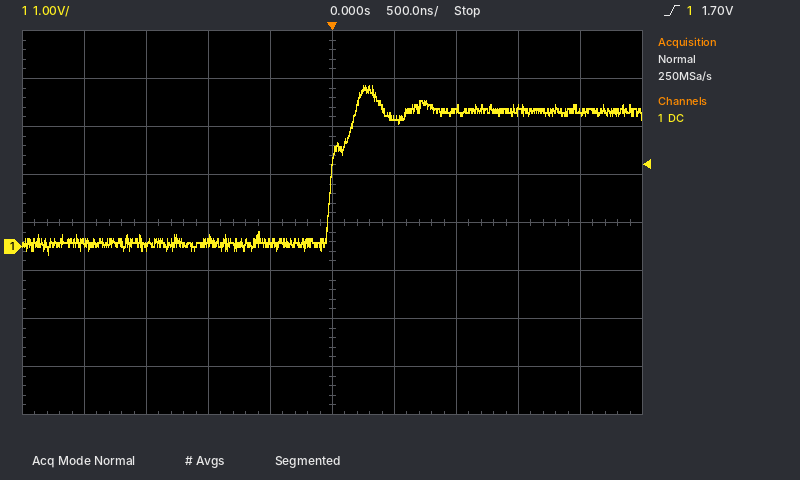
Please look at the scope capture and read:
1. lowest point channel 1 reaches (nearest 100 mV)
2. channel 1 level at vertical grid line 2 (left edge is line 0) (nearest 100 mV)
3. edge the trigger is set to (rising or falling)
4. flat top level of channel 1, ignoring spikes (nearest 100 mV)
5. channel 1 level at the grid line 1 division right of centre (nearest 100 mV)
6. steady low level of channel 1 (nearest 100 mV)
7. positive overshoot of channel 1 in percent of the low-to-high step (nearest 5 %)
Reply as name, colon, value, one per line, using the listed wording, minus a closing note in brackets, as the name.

lowest point channel 1 reaches: -200 mV
channel 1 level at vertical grid line 2 (left edge is line 0): 0.0 V
edge the trigger is set to: rising
flat top level of channel 1, ignoring spikes: 2.8 V
channel 1 level at the grid line 1 division right of centre: 2.7 V
steady low level of channel 1: 100 mV
positive overshoot of channel 1 in percent of the low-to-high step: 20 %
